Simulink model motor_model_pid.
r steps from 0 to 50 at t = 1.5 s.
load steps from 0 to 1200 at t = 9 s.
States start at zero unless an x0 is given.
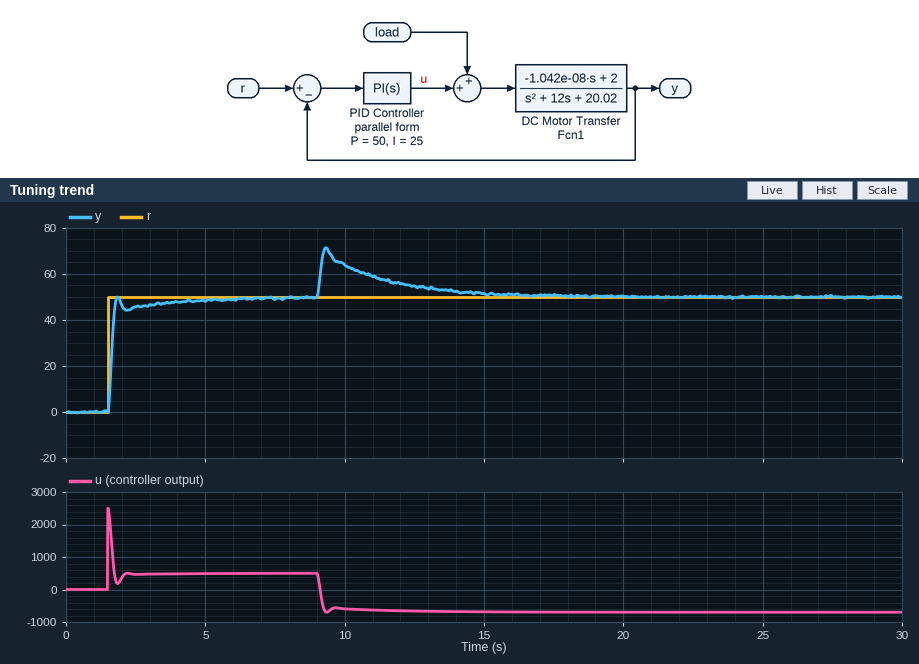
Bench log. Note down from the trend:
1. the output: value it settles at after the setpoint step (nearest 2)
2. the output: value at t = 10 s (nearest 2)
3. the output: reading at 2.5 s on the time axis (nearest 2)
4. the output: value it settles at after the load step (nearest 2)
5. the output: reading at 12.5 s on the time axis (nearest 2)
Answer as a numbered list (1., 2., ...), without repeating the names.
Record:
1. 50
2. 64
3. 46
4. 50
5. 54
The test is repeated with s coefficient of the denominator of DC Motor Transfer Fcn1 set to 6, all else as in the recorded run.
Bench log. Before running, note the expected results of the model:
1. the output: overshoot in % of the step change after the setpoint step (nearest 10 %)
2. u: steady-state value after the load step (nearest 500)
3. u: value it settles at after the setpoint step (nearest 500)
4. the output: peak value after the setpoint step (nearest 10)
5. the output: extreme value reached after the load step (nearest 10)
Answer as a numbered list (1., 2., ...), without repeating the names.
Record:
1. 20 %
2. -500
3. 500
4. 60
5. 80
